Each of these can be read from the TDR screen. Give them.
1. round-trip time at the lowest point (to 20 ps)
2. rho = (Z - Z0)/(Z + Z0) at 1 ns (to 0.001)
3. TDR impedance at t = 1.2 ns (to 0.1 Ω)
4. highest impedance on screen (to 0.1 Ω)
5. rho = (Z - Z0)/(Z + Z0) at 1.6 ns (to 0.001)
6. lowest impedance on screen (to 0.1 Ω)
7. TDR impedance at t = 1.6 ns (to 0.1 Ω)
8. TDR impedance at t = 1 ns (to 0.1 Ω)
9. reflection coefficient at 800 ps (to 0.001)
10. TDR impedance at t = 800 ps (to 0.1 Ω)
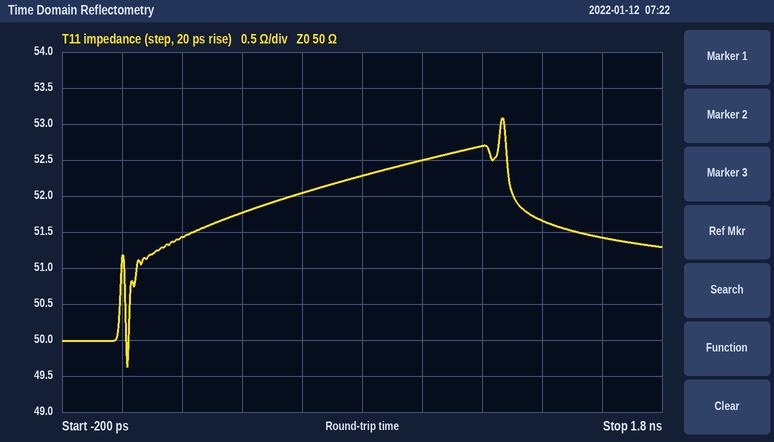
20 ps
+0.024
52.7 Ω
53.1 Ω
+0.014
49.6 Ω
51.4 Ω
52.5 Ω
+0.022
52.3 Ω
